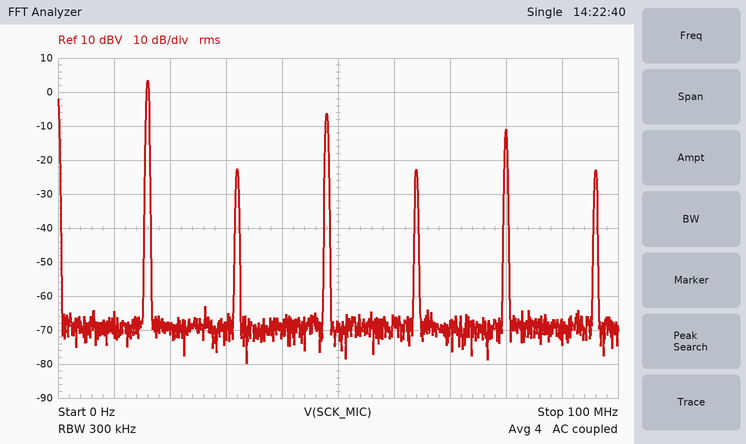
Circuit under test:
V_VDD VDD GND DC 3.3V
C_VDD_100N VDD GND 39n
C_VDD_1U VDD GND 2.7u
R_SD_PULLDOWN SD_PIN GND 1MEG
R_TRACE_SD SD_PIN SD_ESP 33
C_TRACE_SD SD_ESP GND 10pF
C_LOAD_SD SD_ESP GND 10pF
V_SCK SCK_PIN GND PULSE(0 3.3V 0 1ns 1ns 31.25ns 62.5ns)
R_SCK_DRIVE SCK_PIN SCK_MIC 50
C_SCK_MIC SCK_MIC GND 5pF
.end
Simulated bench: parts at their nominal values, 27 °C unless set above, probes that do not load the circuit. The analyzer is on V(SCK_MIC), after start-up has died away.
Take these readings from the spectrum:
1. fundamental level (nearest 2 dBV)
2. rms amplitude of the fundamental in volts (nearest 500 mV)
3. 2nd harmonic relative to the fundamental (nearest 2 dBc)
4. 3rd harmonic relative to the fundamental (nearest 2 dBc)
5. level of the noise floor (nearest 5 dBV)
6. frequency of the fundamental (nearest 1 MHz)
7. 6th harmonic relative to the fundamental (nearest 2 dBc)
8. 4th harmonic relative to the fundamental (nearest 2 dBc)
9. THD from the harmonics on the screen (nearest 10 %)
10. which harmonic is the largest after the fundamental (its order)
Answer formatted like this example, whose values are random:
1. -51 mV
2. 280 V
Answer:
1. 4 dBV
2. 1.5 V
3. -26 dBc
4. -10 dBc
5. -70 dBV
6. 16 MHz
7. -26 dBc
8. -26 dBc
9. 40 %
10. 3
